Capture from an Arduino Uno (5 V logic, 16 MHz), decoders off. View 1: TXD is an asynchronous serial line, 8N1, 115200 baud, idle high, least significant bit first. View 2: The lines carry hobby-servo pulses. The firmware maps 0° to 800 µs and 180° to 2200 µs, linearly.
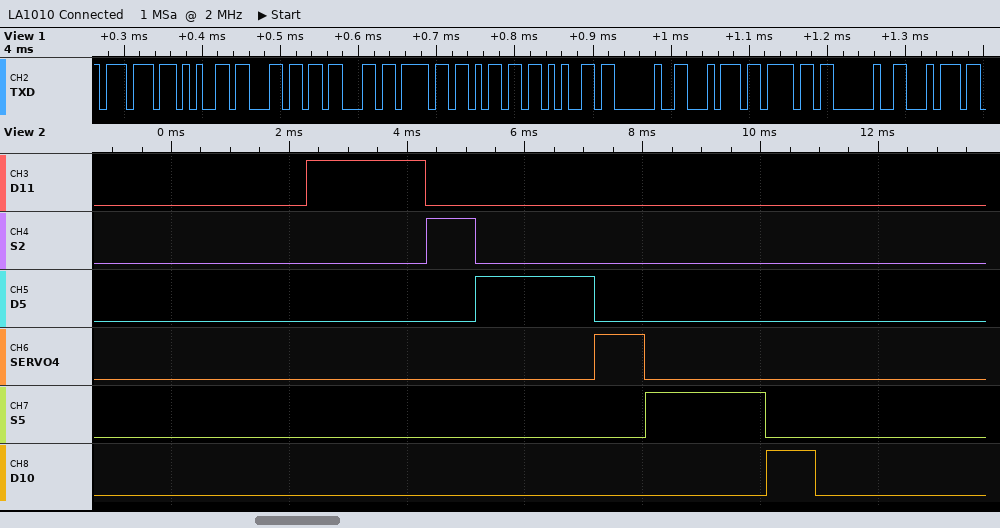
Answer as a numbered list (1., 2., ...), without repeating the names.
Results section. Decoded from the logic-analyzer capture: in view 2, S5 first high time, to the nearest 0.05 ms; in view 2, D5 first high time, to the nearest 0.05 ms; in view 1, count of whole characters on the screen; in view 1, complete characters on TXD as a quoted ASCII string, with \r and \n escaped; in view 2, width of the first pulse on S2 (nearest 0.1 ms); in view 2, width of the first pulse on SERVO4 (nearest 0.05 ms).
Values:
1. 2.05 ms
2. 2.00 ms
3. 12
4. "welcome to t"
5. 0.8 ms
6. 0.85 ms
